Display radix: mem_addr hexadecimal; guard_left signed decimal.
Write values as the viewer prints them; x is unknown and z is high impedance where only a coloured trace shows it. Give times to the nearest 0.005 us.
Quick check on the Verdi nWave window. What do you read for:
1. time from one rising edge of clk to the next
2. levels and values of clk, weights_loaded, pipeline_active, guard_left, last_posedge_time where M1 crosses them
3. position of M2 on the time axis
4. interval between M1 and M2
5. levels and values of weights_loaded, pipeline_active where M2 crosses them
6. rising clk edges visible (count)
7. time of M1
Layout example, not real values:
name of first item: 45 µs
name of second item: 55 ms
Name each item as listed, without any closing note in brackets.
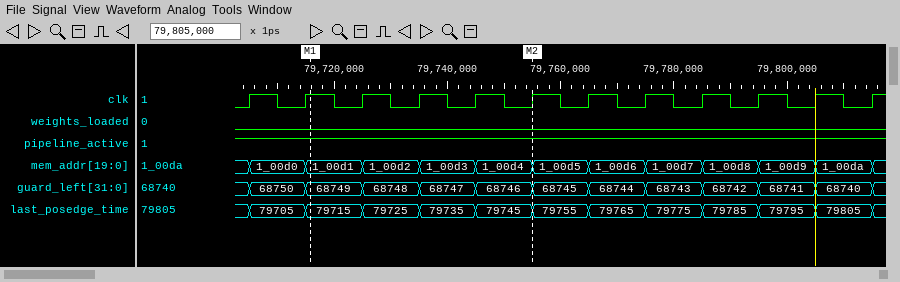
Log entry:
time from one rising edge of clk to the next: 0.01 us
levels and values of clk, weights_loaded, pipeline_active, guard_left, last_posedge_time where M1 crosses them: clk=1, weights_loaded=0, pipeline_active=1, guard_left=68749, last_posedge_time=79715
position of M2 on the time axis: 79.755 us
interval between M1 and M2: 0.04 us
levels and values of weights_loaded, pipeline_active where M2 crosses them: weights_loaded=0, pipeline_active=1
rising clk edges visible: 12
time of M1: 79.715 us
